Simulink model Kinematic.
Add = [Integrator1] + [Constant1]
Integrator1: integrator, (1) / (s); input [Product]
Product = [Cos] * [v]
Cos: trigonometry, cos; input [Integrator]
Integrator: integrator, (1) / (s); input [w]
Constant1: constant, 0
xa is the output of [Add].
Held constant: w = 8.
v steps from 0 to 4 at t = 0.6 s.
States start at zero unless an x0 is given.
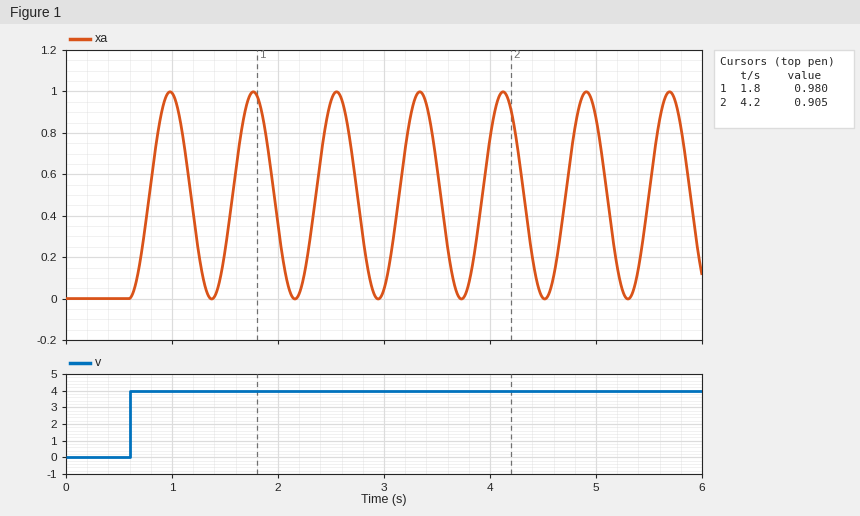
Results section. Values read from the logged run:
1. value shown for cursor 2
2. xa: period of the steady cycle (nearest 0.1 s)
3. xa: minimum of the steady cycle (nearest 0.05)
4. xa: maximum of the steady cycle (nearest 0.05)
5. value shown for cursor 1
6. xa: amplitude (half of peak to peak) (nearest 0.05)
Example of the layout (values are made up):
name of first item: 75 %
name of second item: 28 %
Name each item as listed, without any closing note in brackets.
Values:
value shown for cursor 2: 0.905
xa: period of the steady cycle: 0.8 s
xa: minimum of the steady cycle: 0.00
xa: maximum of the steady cycle: 1.00
value shown for cursor 1: 0.980
xa: amplitude (half of peak to peak): 0.50
